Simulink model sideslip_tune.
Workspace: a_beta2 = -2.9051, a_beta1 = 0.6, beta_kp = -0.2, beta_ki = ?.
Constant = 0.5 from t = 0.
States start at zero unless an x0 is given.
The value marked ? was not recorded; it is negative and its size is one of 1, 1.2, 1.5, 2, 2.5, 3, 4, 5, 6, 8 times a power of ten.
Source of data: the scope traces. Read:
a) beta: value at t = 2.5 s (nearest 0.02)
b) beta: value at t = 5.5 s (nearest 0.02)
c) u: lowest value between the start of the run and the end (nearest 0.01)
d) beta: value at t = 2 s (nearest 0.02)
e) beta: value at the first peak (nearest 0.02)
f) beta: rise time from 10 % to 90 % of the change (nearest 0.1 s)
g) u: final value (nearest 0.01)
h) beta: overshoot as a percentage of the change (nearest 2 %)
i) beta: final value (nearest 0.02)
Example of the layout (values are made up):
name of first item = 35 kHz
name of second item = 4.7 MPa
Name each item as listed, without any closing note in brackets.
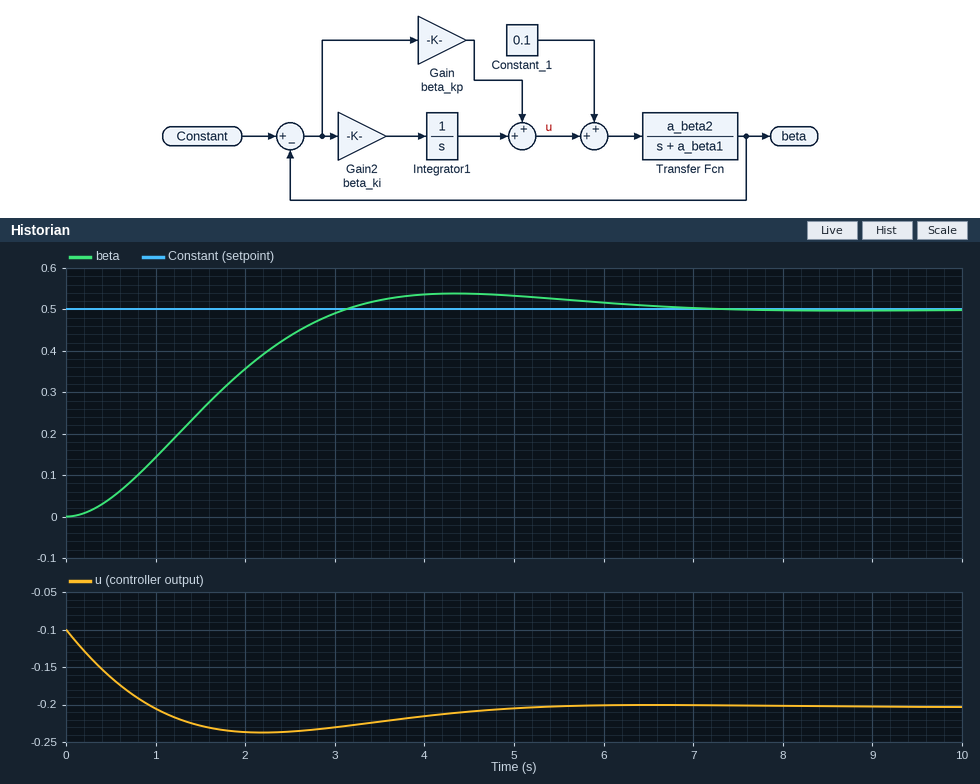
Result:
beta: value at t = 2.5 s = 0.44
beta: value at t = 5.5 s = 0.52
u: lowest value between the start of the run and the end = -0.24
beta: value at t = 2 s = 0.36
beta: value at the first peak = 0.54
beta: rise time from 10 % to 90 % of the change = 2.1 s
u: final value = -0.20
beta: overshoot as a percentage of the change = 8 %
beta: final value = 0.50
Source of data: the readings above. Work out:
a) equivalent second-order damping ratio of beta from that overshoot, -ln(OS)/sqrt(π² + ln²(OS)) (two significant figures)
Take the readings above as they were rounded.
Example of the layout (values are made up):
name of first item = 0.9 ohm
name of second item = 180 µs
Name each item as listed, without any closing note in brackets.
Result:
equivalent second-order damping ratio of beta from that overshoot, -ln(OS)/sqrt(π² + ln²(OS)) = 0.63
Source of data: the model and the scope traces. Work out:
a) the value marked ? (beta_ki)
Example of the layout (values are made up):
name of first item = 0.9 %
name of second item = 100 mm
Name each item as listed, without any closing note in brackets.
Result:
the value marked ? = -0.3
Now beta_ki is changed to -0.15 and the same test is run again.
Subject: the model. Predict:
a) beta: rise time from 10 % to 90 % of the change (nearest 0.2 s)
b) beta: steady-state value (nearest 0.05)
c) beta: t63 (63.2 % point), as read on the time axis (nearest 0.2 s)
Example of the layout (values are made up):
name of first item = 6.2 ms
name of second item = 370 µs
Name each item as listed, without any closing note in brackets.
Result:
beta: rise time from 10 % to 90 % of the change = 4.4 s
beta: steady-state value = 0.50
beta: t63 (63.2 % point), as read on the time axis = 3.0 s
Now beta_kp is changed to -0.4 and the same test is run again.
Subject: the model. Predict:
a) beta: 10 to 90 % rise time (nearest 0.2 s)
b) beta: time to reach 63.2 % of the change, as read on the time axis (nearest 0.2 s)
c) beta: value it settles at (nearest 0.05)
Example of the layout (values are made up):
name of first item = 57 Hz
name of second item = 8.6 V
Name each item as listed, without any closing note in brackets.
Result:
beta: 10 to 90 % rise time = 2.8 s
beta: time to reach 63.2 % of the change, as read on the time axis = 1.4 s
beta: value it settles at = 0.50
